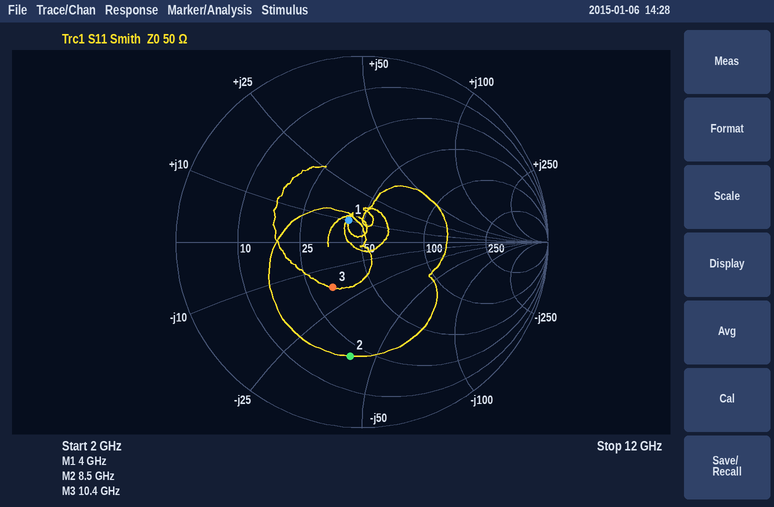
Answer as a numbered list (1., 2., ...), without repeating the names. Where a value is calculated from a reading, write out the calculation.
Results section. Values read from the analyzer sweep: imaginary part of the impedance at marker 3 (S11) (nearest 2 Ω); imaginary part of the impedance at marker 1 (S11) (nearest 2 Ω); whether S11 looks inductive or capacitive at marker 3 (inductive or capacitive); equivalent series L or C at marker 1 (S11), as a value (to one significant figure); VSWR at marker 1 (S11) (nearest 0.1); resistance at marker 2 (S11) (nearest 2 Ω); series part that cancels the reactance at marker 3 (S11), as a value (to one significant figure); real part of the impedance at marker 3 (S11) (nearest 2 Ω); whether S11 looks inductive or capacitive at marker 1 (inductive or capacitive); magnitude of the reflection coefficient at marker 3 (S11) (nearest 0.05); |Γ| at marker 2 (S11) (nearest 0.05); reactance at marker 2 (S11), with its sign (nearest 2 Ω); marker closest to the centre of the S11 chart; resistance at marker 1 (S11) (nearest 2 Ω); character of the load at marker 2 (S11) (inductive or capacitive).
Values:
1. -18 Ω
2. +10 Ω
3. capacitive
4. L = 10 Ω/(2π × 4 GHz) ≈ 398 pH, so 400 pH to one significant figure
5. 1.3
6. 20 Ω
7. L = 18 Ω/(2π × 10.4 GHz) ≈ 275 pH, so 300 pH to one significant figure
8. 32 Ω
9. inductive
10. 0.30
11. 0.60
12. -40 Ω
13. marker 1
14. 42 Ω
15. capacitive
